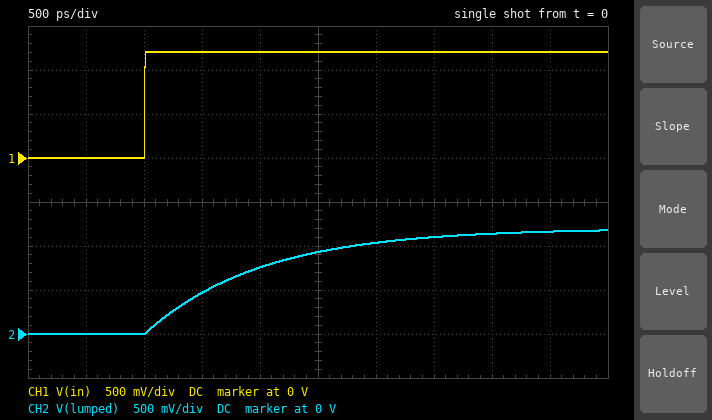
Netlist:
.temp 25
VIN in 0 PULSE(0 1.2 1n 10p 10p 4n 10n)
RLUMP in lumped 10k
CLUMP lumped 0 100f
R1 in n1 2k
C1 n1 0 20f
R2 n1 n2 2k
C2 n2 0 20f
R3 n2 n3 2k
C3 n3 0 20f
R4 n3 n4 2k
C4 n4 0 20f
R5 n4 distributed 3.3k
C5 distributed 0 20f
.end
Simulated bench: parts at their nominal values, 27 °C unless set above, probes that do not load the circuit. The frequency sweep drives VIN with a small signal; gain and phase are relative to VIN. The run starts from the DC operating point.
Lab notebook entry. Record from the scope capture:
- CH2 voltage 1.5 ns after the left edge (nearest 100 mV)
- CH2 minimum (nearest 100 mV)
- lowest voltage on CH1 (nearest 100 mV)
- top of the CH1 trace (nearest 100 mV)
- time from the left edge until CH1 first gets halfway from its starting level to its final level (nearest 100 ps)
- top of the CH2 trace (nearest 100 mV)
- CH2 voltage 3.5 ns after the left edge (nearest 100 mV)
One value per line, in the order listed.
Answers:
500 mV
0 V
0 V
1.2 V
1.0 ns
1.2 V
1.1 V
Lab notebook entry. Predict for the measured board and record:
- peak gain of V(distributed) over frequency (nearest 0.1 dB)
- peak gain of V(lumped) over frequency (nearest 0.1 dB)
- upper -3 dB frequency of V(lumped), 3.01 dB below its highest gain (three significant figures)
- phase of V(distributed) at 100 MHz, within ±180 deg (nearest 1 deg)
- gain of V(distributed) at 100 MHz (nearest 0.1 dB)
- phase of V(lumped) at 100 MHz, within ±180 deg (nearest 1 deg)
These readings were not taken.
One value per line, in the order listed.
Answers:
0 dB
0 dB
159 MHz
-22 deg
-0.4 dB
-32 deg
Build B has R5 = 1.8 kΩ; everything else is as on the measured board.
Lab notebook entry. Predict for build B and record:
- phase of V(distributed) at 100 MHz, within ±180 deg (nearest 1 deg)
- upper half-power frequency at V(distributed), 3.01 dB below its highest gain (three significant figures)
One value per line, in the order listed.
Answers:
-21 deg
318 MHz
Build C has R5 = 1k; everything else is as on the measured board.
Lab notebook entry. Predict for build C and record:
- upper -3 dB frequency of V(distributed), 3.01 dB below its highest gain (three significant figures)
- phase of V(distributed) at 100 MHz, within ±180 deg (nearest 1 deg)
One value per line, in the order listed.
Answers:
322 MHz
-20 deg
